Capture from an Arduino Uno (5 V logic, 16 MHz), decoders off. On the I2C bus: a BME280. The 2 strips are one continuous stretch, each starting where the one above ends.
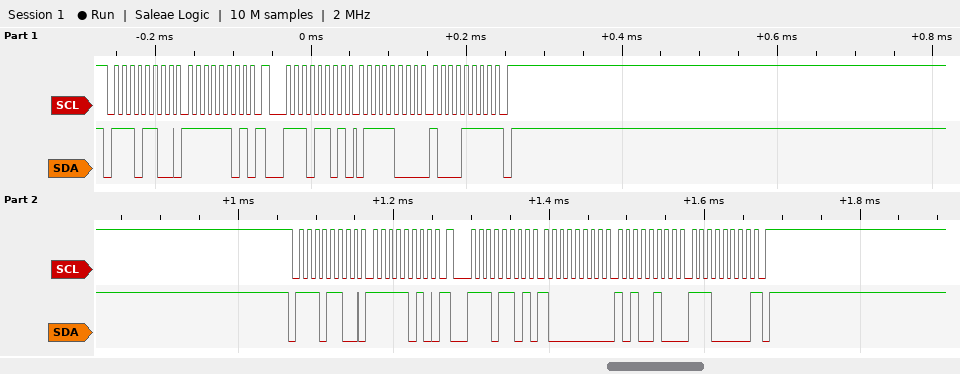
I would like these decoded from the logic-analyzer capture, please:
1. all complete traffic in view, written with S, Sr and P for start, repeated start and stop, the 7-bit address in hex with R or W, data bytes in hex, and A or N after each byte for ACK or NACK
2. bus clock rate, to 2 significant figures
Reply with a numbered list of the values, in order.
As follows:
1. S 76W A FD A Sr 76R A 78 A 8F N P S 76W A FA A Sr 76R A 80 A A4 A E0 N P
2. 100 kHz
